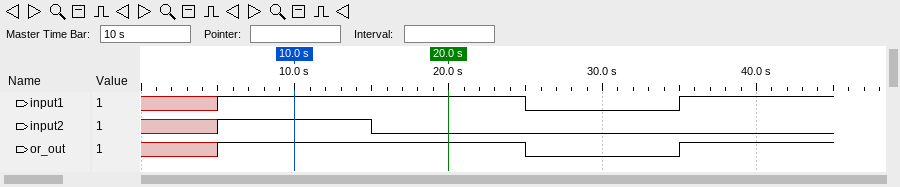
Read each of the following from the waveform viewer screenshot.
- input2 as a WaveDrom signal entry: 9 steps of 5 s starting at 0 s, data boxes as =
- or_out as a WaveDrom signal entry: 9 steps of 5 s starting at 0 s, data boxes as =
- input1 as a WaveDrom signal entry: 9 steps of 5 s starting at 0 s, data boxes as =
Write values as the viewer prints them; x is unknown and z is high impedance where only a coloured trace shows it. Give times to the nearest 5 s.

{name: 'input2', wave: 'x1.0.....'}
{name: 'or_out', wave: 'x1...0.1.'}
{name: 'input1', wave: 'x1...0.1.'}
